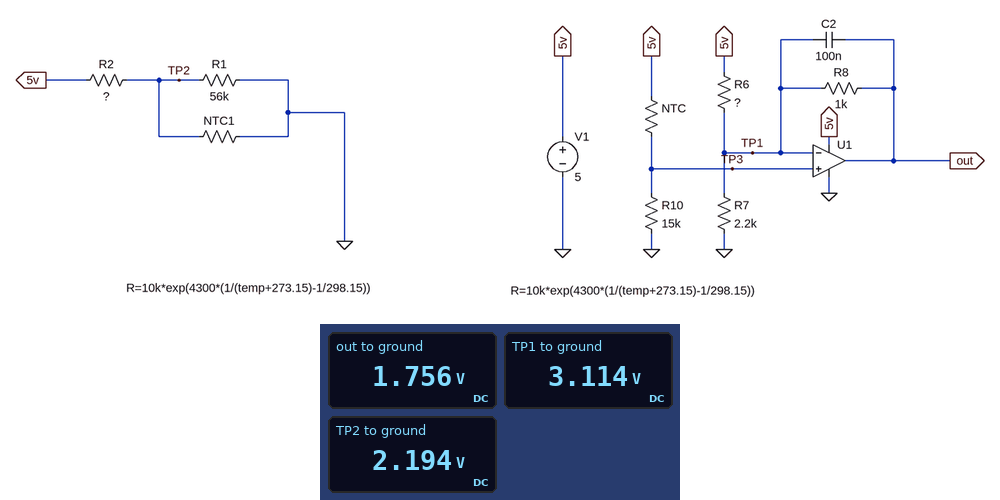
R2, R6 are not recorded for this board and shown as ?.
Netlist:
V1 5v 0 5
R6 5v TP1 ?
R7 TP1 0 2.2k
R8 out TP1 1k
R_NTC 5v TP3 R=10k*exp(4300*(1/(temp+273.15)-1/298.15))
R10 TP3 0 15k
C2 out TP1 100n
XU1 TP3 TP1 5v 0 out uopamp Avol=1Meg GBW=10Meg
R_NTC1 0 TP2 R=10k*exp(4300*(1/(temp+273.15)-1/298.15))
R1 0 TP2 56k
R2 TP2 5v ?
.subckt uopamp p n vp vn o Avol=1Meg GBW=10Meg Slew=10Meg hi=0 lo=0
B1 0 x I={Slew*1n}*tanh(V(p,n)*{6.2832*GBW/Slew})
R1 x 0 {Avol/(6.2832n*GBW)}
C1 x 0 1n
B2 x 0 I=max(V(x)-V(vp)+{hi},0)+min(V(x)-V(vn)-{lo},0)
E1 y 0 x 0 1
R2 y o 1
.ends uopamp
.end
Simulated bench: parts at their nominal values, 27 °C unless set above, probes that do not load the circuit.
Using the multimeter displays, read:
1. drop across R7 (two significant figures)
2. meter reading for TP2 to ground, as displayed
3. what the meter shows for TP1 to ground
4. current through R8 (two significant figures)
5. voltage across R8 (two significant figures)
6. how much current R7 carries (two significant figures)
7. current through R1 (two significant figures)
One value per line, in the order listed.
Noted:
3.1 V
2.194 V
3.114 V
1.4 mA
1.4 V
1.4 mA
39 µA
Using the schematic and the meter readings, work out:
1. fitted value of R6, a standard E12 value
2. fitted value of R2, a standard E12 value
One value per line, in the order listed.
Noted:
680 Ω
10 kΩ
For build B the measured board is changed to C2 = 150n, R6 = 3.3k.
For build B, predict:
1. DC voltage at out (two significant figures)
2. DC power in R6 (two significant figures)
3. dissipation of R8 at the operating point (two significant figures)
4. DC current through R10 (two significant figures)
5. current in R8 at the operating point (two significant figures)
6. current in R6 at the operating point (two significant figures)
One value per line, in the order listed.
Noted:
4.0 V
1.1 mW
710 µW
210 µA
840 µA
570 µA
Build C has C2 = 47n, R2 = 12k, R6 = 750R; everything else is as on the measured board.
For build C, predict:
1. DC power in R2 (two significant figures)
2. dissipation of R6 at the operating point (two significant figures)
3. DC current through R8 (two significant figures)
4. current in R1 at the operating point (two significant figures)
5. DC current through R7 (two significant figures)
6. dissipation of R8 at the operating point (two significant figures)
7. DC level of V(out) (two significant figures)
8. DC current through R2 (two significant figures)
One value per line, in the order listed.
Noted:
760 µW
4.7 mW
1.1 mA
35 µA
1.4 mA
1.2 mW
2.0 V
250 µA
